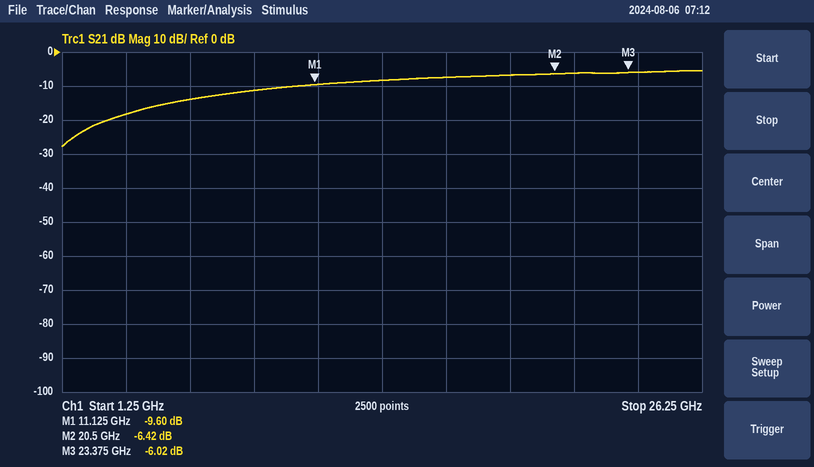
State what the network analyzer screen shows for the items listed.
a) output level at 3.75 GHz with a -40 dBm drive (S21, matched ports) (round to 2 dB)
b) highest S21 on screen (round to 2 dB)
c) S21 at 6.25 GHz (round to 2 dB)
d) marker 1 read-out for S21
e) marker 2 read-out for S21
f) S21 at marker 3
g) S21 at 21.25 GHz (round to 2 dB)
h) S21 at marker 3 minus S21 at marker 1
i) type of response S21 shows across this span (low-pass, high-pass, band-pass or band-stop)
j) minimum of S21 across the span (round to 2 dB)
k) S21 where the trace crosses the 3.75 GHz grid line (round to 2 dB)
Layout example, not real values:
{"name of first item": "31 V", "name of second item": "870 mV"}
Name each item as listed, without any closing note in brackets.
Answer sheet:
{"output level at 3.75 GHz with a -40 dBm drive (S21, matched ports)": "-58 dBm", "highest S21 on screen": "-6 dB", "S21 at 6.25 GHz": "-14 dB", "marker 1 read-out for S21": "-9.60 dB", "marker 2 read-out for S21": "-6.42 dB", "S21 at marker 3": "-6.02 dB", "S21 at 21.25 GHz": "-6 dB", "S21 at marker 3 minus S21 at marker 1": "3.58 dB", "type of response S21 shows across this span": "high-pass", "minimum of S21 across the span": "-28 dB", "S21 where the trace crosses the 3.75 GHz grid line": "-18 dB"}
